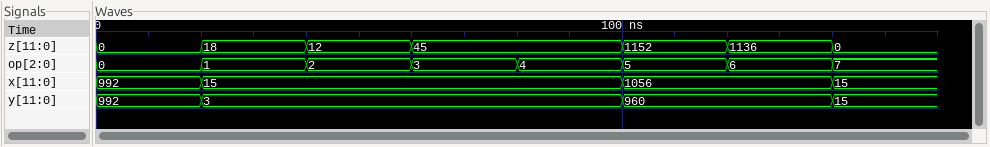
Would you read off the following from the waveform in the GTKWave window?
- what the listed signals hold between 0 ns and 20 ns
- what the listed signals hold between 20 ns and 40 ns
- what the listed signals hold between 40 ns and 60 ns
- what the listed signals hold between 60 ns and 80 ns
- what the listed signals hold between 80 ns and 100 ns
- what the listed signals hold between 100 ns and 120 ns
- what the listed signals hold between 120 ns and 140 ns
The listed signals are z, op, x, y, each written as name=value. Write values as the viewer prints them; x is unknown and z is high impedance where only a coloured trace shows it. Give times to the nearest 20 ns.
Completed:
z=0, op=0, x=992, y=992
z=18, op=1, x=15, y=3
z=12, op=2, x=15, y=3
z=45, op=3, x=15, y=3
z=45, op=4, x=15, y=3
z=1152, op=5, x=1056, y=960
z=1136, op=6, x=1056, y=960
